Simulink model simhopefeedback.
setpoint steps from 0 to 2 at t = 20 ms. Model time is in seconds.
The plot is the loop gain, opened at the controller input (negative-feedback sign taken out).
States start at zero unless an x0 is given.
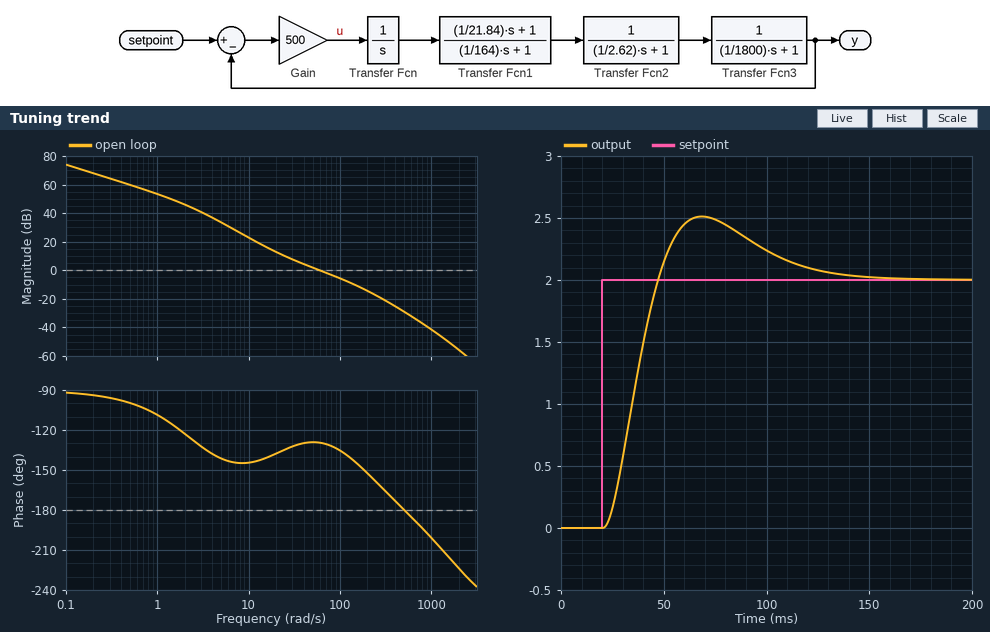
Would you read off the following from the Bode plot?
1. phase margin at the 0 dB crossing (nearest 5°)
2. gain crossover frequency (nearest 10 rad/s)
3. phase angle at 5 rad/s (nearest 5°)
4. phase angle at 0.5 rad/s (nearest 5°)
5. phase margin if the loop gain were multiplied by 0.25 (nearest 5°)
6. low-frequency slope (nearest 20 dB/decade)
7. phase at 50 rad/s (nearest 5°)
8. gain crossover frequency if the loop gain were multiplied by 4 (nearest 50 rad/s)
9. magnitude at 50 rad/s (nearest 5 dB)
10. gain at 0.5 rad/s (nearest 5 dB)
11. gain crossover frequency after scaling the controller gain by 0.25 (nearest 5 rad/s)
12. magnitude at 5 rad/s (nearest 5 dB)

50°
60 rad/s
-140°
-100°
45°
-20 dB/decade
-130°
150 rad/s
0 dB
60 dB
20 rad/s
35 dB
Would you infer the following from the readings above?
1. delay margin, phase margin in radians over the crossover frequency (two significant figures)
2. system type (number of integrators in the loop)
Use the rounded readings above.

0.015 s
1
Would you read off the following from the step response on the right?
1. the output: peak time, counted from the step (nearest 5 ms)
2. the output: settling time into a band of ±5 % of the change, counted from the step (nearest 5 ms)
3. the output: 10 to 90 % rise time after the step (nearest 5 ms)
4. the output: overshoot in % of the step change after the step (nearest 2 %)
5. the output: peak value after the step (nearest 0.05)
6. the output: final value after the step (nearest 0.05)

50 ms
100 ms
20 ms
26 %
2.50
2.00
